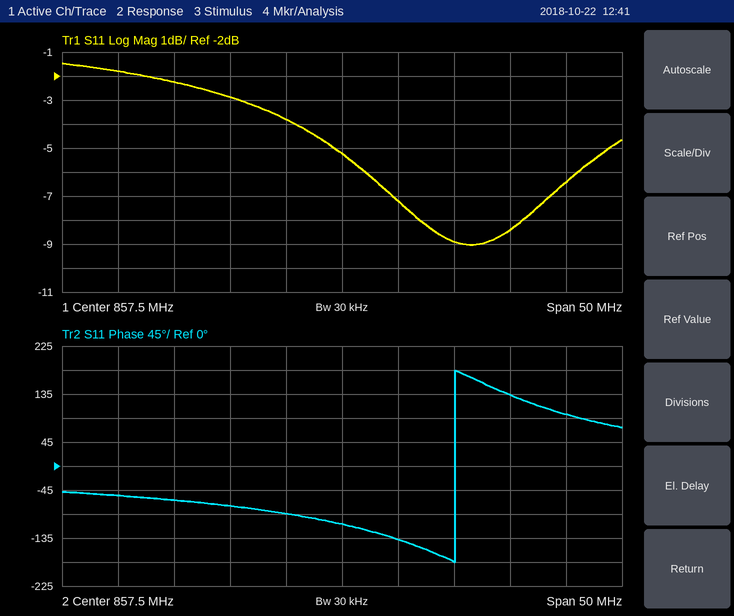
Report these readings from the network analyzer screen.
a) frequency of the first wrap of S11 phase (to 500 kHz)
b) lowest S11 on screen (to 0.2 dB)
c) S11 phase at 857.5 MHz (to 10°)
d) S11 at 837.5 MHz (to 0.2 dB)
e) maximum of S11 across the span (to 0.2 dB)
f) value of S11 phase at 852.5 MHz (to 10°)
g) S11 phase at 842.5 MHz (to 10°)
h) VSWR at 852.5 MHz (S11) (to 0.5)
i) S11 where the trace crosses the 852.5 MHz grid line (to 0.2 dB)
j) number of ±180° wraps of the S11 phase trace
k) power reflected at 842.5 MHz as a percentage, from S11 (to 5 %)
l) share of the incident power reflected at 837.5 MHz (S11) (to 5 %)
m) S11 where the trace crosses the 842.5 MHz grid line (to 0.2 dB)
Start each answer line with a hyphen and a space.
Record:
- 867.5 MHz
- -9.0 dB
- -110°
- -1.8 dB
- -1.4 dB
- -90°
- -60°
- 4.5
- -3.8 dB
- 1
- 60 %
- 65 %
- -2.2 dB
